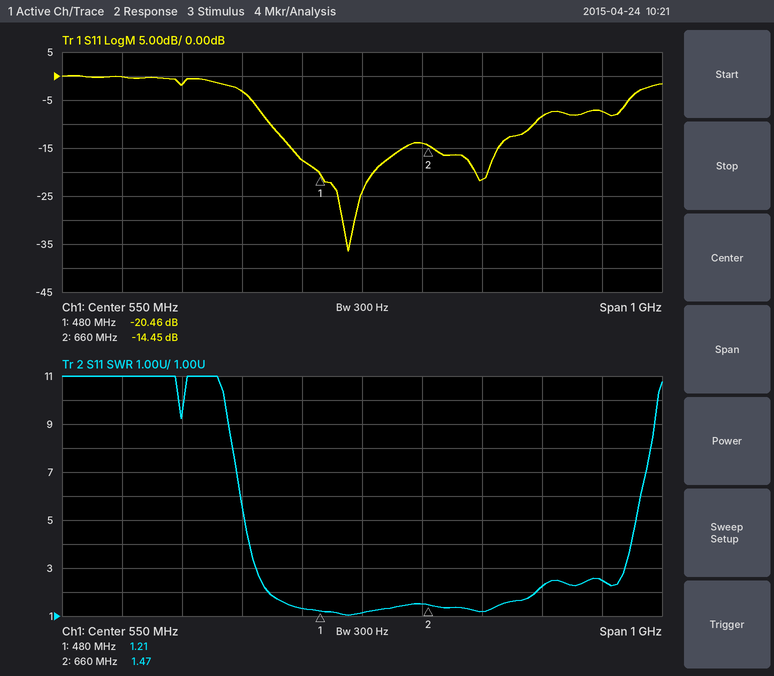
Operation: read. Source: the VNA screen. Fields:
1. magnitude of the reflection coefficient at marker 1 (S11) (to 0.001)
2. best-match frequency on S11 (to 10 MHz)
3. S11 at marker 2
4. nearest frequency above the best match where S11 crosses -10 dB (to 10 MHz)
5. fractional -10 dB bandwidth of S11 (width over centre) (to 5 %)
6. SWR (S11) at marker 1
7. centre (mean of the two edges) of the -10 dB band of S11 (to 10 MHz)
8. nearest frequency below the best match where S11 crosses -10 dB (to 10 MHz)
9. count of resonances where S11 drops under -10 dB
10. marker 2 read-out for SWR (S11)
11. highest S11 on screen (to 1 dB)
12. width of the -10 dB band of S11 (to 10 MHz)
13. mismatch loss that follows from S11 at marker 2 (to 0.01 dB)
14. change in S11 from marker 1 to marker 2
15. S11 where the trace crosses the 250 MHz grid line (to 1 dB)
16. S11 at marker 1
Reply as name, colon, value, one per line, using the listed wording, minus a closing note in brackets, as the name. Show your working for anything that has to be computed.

magnitude of the reflection coefficient at marker 1 (S11): 10^(-20.46/20) ≈ 0.095
best-match frequency on S11: 530 MHz
S11 at marker 2: -14.45 dB
nearest frequency above the best match where S11 crosses -10 dB: 840 MHz
fractional -10 dB bandwidth of S11 (width over centre): 440 MHz / 620 MHz ≈ 71.0 %, so 70 % to the nearest 5 %
SWR (S11) at marker 1: 1.21
centre (mean of the two edges) of the -10 dB band of S11: 620 MHz
nearest frequency below the best match where S11 crosses -10 dB: 400 MHz
count of resonances where S11 drops under -10 dB: 2
marker 2 read-out for SWR: 1.47
highest S11 on screen: 0 dB
width of the -10 dB band of S11: 840 MHz − 400 MHz = 440 MHz
mismatch loss that follows from S11 at marker 2: −10 log10(1 − 10^(-14.45/10)) ≈ 0.16 dB
change in S11 from marker 1 to marker 2: -14.45 − (-20.46) = 6.01 dB
S11 where the trace crosses the 250 MHz grid line: -2 dB
S11 at marker 1: -20.46 dB
